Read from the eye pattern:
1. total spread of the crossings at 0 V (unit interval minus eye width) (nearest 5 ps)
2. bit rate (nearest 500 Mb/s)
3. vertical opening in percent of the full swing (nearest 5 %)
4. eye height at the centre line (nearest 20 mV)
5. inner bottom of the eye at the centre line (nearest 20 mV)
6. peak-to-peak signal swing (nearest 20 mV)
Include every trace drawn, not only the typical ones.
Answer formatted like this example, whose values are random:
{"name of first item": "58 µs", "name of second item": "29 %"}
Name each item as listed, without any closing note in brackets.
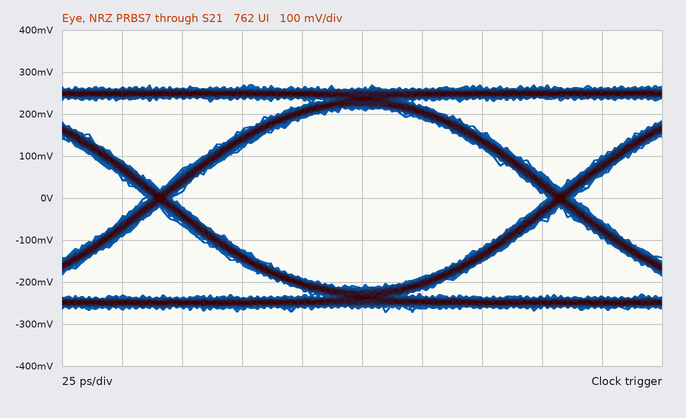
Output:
{"total spread of the crossings at 0 V (unit interval minus eye width)": "10 ps", "bit rate": "6.0 Gb/s", "vertical opening in percent of the full swing": "80 %", "eye height at the centre line": "420 mV", "inner bottom of the eye at the centre line": "-220 mV", "peak-to-peak signal swing": "540 mV"}
